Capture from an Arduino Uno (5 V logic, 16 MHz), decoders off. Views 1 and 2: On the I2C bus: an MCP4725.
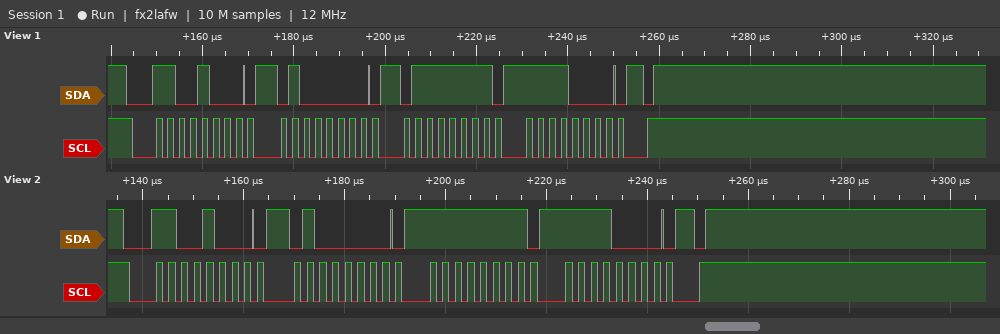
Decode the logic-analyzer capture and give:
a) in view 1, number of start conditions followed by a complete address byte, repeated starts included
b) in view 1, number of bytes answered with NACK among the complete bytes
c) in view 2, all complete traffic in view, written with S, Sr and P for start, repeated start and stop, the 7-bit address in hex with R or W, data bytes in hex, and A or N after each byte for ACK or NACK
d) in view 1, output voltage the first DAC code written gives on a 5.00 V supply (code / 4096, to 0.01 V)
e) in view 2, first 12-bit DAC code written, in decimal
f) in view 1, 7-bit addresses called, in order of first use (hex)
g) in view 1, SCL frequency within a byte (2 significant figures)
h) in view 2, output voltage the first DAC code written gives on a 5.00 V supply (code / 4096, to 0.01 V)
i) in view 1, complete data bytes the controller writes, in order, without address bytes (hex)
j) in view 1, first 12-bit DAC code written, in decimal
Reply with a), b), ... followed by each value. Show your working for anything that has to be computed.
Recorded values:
a) 1
b) 0
c) S 64W A 40 A FF A F0 A P
d) 2047 / 4096 x 5.00 V = 2.50 V
e) 4095
f) 0x64
g) 400 kHz
h) 4095 / 4096 x 5.00 V = 5.00 V
i) 40 7F F0
j) 2047
